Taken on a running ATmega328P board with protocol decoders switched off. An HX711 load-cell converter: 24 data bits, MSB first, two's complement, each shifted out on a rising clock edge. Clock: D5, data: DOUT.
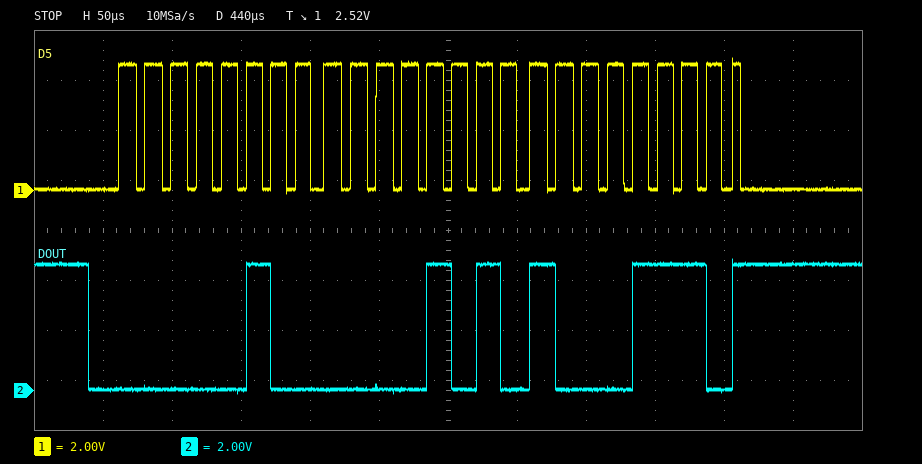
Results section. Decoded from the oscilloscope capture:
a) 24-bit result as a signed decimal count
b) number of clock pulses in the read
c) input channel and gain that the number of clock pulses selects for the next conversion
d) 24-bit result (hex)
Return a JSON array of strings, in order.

["264846", "25", "channel A, gain 128", "0x040A8E"]
